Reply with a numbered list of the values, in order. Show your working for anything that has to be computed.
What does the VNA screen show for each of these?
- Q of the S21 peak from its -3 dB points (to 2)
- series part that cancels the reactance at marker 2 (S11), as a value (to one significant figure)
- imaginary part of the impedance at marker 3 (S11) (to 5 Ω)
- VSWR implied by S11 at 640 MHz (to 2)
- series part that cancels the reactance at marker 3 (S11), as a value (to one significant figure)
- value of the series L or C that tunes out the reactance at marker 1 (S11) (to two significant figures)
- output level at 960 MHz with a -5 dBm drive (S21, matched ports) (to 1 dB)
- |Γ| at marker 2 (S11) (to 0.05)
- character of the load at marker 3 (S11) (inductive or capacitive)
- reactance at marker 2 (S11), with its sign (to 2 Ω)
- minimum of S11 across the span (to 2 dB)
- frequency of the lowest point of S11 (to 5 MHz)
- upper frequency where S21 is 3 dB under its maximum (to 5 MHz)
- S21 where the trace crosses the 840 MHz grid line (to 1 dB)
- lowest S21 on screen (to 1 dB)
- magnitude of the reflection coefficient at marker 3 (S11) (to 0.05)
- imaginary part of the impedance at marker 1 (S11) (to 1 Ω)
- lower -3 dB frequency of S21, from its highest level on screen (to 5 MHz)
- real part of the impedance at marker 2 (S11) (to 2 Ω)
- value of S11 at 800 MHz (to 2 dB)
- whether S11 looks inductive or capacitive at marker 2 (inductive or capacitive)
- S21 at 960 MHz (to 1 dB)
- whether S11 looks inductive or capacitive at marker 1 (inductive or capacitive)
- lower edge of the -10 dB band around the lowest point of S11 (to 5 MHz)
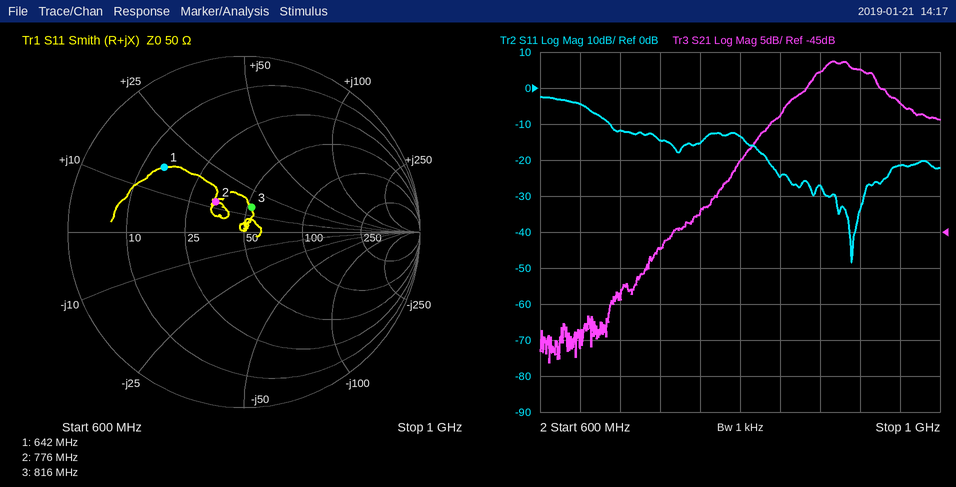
1. 902.5 MHz / 65 MHz ≈ 14
2. C = 1/(2π × 776 MHz × 12 Ω) ≈ 17.1 pF, so 20 pF to one significant figure
3. +15 Ω
4. |Γ| = 10^(-4/20) = 0.6310; VSWR = (1 + 0.6310)/(1 − 0.6310) ≈ 4
5. C = 1/(2π × 816 MHz × 15 Ω) ≈ 13.0 pF, so 10 pF to one significant figure
6. C = 1/(2π × 642 MHz × 16 Ω) ≈ 15 pF
7. -5 dBm + (-27 dB) = -32 dBm
8. 0.25
9. inductive
10. +12 Ω
11. -48 dB
12. 910 MHz
13. 935 MHz
14. -29 dB
15. -63 dB
16. 0.15
17. +16 Ω
18. 870 MHz
19. 34 Ω
20. -14 dB
21. inductive
22. -27 dB
23. inductive
24. 670 MHz
